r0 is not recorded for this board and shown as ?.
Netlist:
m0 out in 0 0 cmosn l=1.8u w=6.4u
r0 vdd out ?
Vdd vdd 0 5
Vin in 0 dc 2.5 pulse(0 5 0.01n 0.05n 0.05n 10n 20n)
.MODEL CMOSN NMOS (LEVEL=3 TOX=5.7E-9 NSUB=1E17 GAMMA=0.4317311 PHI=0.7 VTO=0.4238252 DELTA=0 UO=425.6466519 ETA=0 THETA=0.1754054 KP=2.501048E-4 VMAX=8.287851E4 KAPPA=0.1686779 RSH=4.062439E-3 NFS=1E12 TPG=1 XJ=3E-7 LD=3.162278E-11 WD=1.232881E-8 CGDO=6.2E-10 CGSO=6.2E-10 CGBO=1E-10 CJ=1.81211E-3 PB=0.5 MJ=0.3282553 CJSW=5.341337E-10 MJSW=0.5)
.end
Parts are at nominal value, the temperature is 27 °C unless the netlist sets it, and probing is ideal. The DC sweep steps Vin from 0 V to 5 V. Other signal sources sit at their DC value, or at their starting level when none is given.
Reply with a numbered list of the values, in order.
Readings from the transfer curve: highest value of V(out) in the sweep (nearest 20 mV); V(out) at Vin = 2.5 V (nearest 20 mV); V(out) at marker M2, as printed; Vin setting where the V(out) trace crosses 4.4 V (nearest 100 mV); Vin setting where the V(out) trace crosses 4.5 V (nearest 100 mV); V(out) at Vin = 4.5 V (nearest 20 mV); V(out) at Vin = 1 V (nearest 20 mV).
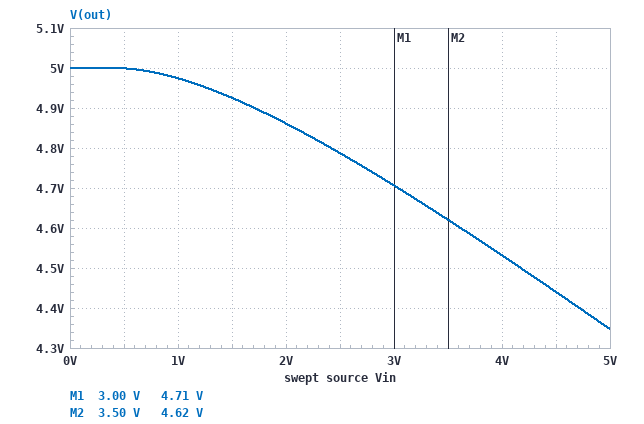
1. 5.00 V
2. 4.78 V
3. 4.62 V
4. 4.7 V
5. 4.2 V
6. 4.44 V
7. 4.98 V
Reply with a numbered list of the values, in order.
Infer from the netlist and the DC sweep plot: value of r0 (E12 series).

1. 220 Ω
